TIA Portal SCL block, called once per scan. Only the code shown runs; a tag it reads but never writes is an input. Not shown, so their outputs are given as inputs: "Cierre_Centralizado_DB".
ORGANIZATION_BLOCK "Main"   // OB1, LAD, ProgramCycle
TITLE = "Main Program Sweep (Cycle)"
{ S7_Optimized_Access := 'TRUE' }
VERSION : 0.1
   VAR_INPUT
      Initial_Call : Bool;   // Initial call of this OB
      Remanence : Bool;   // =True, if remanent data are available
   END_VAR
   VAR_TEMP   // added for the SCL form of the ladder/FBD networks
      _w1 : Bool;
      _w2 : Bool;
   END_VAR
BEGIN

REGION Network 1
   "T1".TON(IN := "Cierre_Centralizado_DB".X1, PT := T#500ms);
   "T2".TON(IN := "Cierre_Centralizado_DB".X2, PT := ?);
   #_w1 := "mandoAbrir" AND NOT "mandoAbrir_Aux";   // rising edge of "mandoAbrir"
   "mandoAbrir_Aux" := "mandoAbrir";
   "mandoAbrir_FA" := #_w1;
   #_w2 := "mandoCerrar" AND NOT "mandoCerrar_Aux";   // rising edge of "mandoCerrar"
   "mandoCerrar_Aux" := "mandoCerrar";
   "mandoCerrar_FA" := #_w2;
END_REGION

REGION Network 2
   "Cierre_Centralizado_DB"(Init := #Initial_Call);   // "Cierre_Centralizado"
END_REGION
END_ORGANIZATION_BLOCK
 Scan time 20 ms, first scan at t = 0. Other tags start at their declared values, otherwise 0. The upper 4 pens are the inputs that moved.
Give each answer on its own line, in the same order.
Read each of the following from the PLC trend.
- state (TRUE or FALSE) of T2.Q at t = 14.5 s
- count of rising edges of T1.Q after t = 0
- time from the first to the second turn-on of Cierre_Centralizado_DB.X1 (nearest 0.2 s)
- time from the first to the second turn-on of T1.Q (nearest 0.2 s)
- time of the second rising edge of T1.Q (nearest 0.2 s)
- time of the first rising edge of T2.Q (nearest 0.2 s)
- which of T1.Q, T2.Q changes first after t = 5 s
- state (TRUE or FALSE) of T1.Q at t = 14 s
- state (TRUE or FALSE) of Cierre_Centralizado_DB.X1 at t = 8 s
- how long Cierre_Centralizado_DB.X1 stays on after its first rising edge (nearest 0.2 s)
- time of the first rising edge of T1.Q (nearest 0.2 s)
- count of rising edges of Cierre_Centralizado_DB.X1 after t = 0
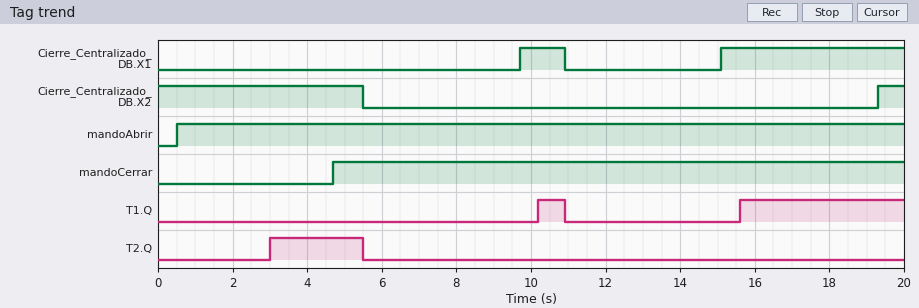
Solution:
FALSE
2
5.4 s
5.4 s
15.6 s
3.0 s
T2.Q
FALSE
FALSE
1.2 s
10.2 s
2
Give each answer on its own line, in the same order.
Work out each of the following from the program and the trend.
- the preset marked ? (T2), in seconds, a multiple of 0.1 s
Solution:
3.0 s
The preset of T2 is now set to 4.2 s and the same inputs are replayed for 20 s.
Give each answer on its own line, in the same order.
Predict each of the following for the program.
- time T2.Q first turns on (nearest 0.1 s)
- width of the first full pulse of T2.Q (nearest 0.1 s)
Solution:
4.2 s
1.3 s
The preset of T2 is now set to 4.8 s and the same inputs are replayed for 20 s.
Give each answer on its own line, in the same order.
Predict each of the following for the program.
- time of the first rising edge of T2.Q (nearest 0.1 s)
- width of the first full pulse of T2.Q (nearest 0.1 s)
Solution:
4.8 s
0.7 s
